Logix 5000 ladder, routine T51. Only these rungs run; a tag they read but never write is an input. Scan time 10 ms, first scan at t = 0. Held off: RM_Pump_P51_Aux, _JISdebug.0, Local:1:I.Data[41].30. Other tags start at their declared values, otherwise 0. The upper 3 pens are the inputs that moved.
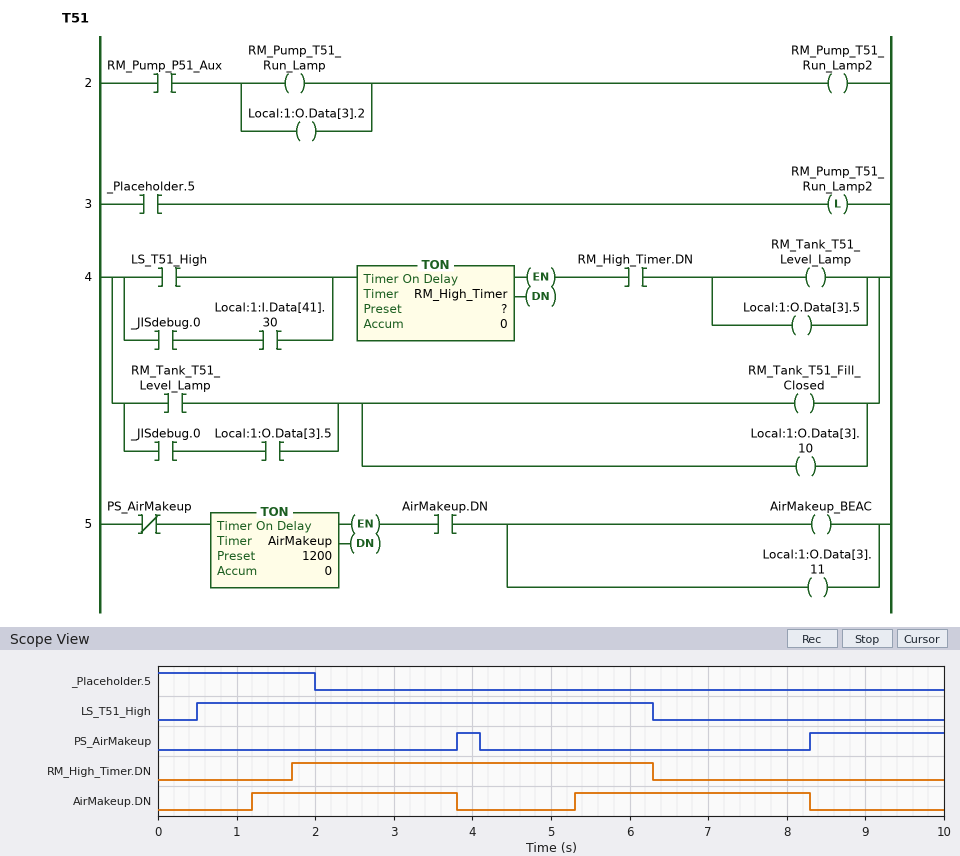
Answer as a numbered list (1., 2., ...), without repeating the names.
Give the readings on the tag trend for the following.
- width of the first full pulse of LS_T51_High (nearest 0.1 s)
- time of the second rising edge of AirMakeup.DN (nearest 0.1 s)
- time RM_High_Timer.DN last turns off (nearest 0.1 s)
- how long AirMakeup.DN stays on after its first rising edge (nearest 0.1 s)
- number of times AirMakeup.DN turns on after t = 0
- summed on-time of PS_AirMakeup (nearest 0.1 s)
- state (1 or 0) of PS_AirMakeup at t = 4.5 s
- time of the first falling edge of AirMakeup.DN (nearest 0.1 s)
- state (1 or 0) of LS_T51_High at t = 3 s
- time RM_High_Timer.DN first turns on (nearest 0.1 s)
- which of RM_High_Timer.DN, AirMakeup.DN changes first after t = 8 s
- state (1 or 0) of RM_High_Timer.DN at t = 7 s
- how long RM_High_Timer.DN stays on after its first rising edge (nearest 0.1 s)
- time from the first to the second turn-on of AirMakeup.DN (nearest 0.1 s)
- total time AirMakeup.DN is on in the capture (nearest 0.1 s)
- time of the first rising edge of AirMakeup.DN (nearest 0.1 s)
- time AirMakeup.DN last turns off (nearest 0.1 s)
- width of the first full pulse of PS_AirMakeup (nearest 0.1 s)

1. 5.8 s
2. 5.3 s
3. 6.3 s
4. 2.6 s
5. 2
6. 2.0 s
7. 0
8. 3.8 s
9. 1
10. 1.7 s
11. AirMakeup.DN
12. 0
13. 4.6 s
14. 4.1 s
15. 5.6 s
16. 1.2 s
17. 8.3 s
18. 0.3 s
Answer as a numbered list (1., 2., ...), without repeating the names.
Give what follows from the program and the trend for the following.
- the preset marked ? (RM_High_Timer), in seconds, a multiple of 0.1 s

1. 1.2 s
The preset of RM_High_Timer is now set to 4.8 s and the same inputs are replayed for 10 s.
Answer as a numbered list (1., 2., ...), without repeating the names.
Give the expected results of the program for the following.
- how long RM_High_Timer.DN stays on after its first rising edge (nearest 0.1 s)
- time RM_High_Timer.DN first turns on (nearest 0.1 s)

1. 1.0 s
2. 5.3 s
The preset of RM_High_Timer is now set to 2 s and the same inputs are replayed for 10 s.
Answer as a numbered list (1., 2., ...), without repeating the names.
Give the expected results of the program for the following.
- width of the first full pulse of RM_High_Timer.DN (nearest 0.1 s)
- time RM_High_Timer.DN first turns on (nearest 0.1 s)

1. 3.8 s
2. 2.5 s
